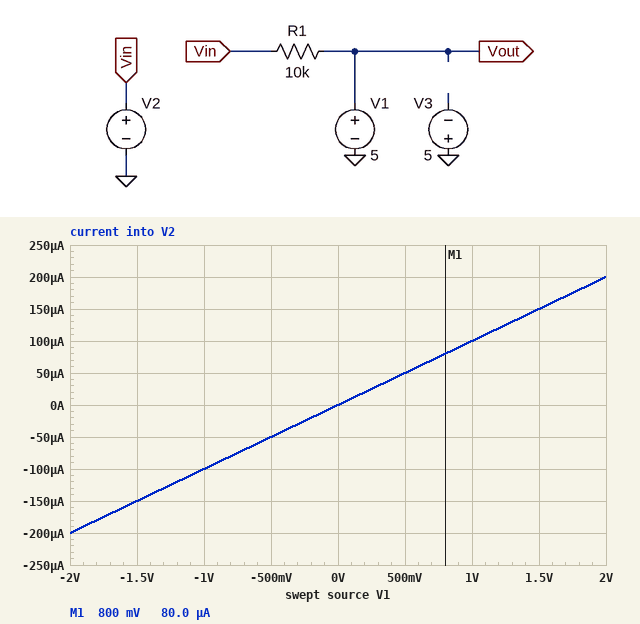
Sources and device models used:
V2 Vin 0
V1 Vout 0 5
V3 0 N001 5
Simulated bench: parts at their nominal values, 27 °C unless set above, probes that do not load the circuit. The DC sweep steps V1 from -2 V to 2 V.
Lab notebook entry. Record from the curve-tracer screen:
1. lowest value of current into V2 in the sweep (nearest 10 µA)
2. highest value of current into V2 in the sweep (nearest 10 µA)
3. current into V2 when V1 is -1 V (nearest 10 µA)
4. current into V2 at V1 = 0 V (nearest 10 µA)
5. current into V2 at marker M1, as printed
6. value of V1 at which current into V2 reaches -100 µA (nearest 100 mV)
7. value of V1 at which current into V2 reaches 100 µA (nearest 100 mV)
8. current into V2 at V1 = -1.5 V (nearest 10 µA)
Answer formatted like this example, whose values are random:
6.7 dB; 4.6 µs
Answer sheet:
-200 µA; 200 µA; -100 µA; 0 A; 80.0 µA; -1.0 V; 1.0 V; -150 µA
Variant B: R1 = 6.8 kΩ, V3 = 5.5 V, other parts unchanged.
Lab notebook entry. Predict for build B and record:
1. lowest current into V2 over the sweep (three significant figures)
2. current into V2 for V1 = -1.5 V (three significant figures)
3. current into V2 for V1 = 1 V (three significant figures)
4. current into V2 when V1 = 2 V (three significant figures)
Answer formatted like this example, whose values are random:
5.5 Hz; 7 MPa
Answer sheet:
-294 µA; -221 µA; 147 µA; 294 µA
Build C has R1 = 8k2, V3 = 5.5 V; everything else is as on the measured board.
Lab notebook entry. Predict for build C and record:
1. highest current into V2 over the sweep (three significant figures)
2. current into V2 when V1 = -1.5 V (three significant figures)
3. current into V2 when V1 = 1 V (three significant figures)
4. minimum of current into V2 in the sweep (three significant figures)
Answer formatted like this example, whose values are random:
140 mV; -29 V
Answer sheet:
244 µA; -183 µA; 122 µA; -244 µA
